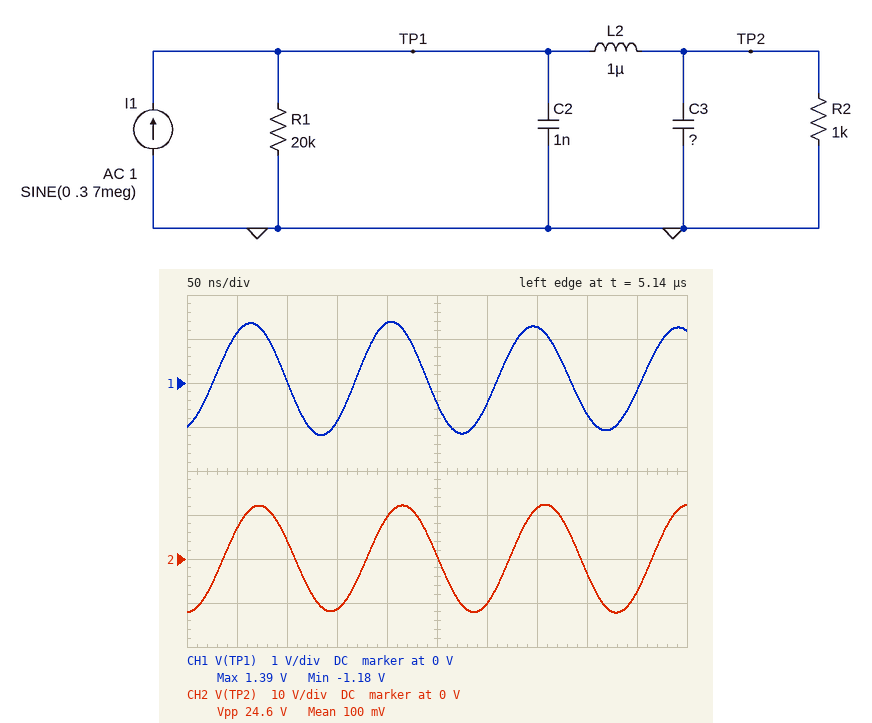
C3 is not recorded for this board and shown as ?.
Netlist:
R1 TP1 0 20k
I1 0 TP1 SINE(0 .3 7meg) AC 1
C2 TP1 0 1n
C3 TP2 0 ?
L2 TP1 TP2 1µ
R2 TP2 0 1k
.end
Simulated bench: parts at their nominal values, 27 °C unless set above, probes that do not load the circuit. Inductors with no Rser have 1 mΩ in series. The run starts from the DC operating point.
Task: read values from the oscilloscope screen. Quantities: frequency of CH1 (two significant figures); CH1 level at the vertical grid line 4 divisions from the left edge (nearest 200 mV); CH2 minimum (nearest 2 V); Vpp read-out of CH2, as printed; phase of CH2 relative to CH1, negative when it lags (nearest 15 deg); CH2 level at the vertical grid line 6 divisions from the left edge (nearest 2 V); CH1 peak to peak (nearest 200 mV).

7.0 MHz
1.4 V
-12 V
24.6 V
-30 deg
-10 V
2.6 V
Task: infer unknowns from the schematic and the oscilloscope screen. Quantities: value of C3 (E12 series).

470 pF
